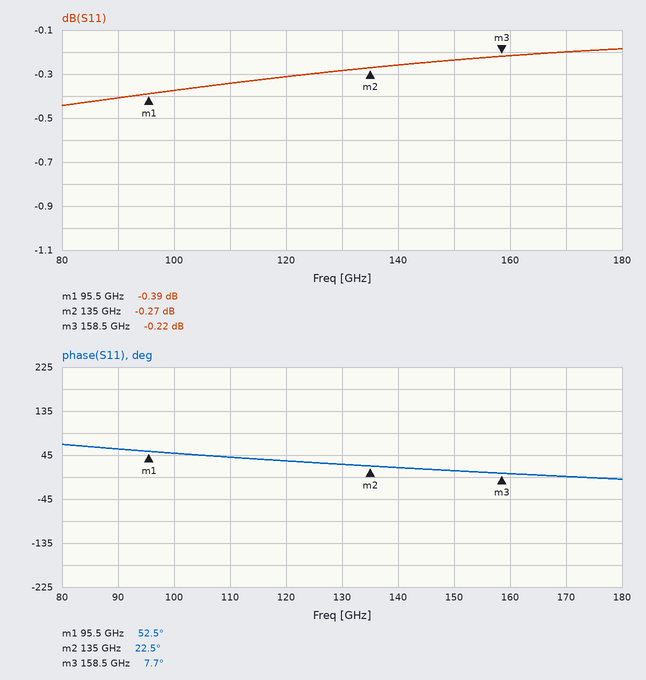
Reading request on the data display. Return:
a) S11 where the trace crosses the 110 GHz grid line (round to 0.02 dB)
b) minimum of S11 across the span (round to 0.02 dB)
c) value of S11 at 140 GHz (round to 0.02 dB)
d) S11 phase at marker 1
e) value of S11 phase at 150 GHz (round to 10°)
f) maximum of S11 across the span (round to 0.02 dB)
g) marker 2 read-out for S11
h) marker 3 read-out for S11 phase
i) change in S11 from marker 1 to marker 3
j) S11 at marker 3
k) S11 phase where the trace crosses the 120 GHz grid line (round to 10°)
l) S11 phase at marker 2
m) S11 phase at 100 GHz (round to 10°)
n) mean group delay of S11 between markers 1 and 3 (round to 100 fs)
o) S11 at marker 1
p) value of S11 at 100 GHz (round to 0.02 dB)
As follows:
-0.34 dB
-0.44 dB
-0.26 dB
52.5°
10°
-0.18 dB
-0.27 dB
7.7°
0.17 dB
-0.22 dB
30°
22.5°
50°
2.0 ps
-0.39 dB
-0.38 dB
